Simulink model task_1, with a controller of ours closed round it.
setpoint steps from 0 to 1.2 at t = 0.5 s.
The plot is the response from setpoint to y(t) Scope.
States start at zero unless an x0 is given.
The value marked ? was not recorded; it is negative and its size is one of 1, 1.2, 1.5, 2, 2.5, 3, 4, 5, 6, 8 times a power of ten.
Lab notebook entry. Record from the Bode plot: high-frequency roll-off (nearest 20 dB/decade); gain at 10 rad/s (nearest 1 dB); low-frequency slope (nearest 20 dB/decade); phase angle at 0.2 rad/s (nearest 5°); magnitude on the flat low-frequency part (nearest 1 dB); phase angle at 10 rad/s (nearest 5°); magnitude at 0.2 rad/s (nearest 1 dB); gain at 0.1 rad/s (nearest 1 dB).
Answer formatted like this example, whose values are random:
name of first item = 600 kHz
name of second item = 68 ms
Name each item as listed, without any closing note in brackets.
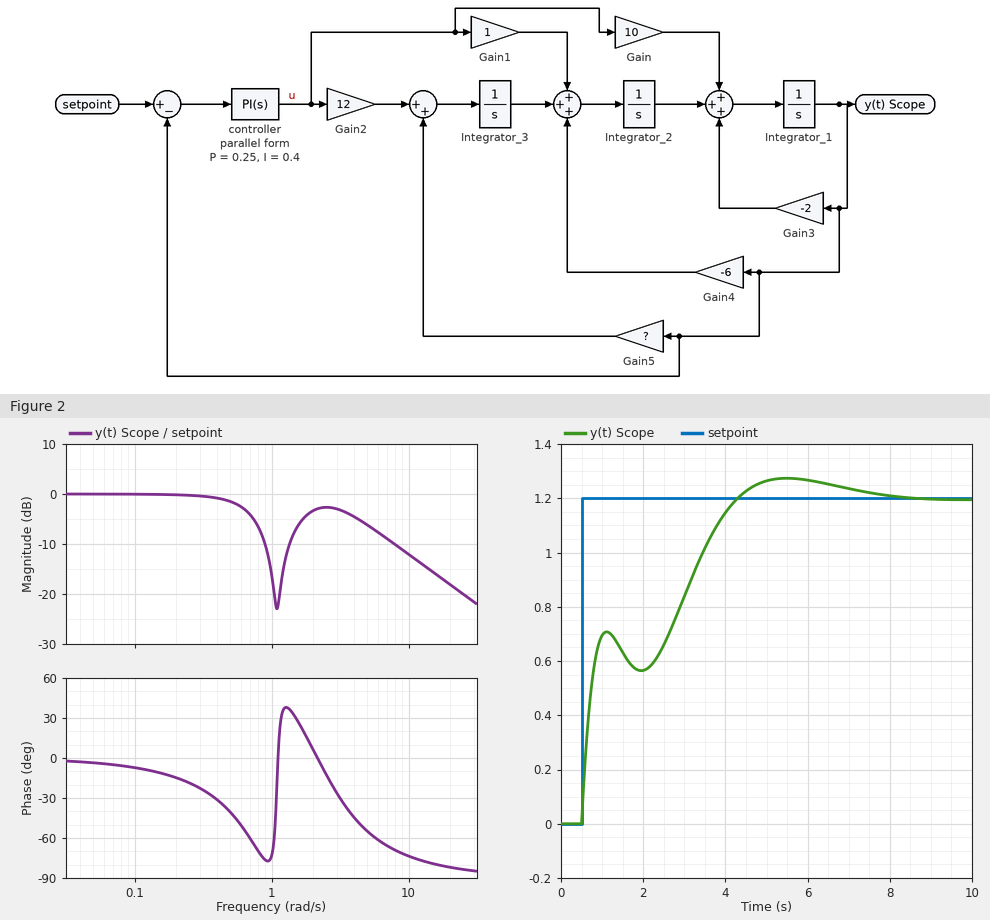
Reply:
high-frequency roll-off = -20 dB/decade
gain at 10 rad/s = -12 dB
low-frequency slope = 0 dB/decade
phase angle at 0.2 rad/s = -15°
magnitude on the flat low-frequency part = 0 dB
phase angle at 10 rad/s = -75°
magnitude at 0.2 rad/s = 0 dB
gain at 0.1 rad/s = 0 dB
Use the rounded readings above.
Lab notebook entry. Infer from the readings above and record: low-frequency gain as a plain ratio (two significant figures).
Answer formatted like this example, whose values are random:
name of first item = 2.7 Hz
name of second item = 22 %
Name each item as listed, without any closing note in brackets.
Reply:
low-frequency gain as a plain ratio = 1.0
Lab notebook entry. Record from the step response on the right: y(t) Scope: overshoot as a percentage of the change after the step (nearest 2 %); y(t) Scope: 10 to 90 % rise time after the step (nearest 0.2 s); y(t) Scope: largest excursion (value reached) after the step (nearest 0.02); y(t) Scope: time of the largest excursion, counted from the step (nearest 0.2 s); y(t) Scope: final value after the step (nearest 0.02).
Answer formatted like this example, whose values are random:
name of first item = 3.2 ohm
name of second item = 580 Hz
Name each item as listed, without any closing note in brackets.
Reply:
y(t) Scope: overshoot as a percentage of the change after the step = 6 %
y(t) Scope: 10 to 90 % rise time after the step = 3.2 s
y(t) Scope: largest excursion (value reached) after the step = 1.28
y(t) Scope: time of the largest excursion, counted from the step = 5.0 s
y(t) Scope: final value after the step = 1.20
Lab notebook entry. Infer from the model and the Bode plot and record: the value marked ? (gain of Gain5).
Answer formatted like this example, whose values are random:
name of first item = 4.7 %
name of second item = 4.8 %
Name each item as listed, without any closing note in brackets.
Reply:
the value marked ? = -6
